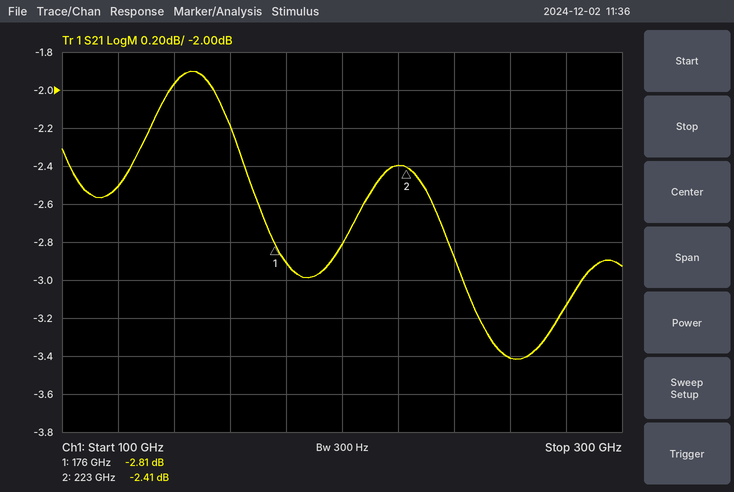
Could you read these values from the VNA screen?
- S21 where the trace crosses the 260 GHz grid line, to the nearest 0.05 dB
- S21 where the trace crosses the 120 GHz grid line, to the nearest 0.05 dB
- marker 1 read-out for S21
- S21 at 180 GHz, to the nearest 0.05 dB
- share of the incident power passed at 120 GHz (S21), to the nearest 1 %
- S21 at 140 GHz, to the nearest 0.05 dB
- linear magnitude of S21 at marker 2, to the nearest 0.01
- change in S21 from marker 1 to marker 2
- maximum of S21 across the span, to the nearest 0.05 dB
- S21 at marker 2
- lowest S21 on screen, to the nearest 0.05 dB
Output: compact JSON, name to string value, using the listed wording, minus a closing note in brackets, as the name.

{"S21 where the trace crosses the 260 GHz grid line, to the nearest 0.05 dB": "-3.40 dB", "S21 where the trace crosses the 120 GHz grid line, to the nearest 0.05 dB": "-2.50 dB", "marker 1 read-out for S21": "-2.81 dB", "S21 at 180 GHz, to the nearest 0.05 dB": "-2.90 dB", "share of the incident power passed at 120 GHz (S21), to the nearest 1 %": "56 %", "S21 at 140 GHz, to the nearest 0.05 dB": "-1.95 dB", "linear magnitude of S21 at marker 2, to the nearest 0.01": "0.76", "change in S21 from marker 1 to marker 2": "0.40 dB", "maximum of S21 across the span, to the nearest 0.05 dB": "-1.90 dB", "S21 at marker 2": "-2.41 dB", "lowest S21 on screen, to the nearest 0.05 dB": "-3.40 dB"}
